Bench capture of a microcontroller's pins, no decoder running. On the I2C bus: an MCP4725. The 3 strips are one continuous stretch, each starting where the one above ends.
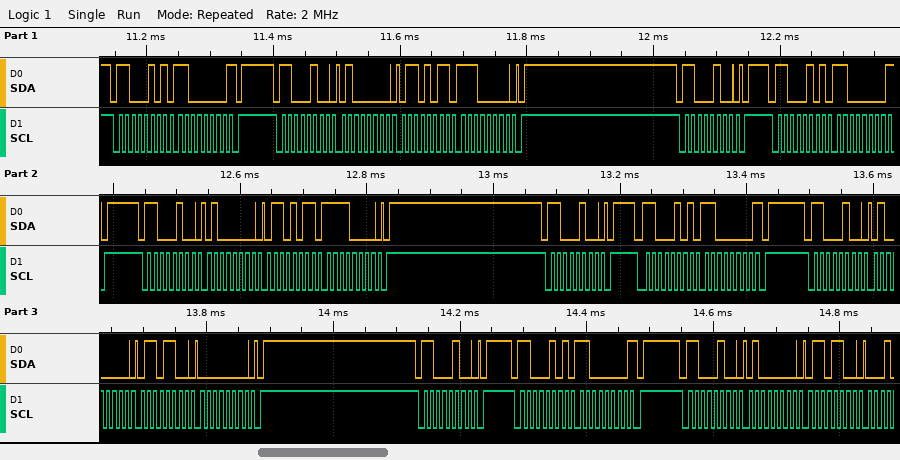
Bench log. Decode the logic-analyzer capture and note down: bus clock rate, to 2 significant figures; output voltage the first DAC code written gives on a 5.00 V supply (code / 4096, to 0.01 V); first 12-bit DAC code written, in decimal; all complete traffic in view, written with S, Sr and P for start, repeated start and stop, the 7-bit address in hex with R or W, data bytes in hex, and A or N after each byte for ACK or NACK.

100 kHz
2.11 V
1726
S 62R A C0 N P S 62W A 40 A 6B A E0 A P S 62W A P S 62R A C0 N P S 62W A 40 A 6B A F0 A P S 62W A P S 62R A C0 N P S 62W A 40 A 6C A 00 A P S 62W A P S 62R A C0 N P S 62W A 40 A 6C A
